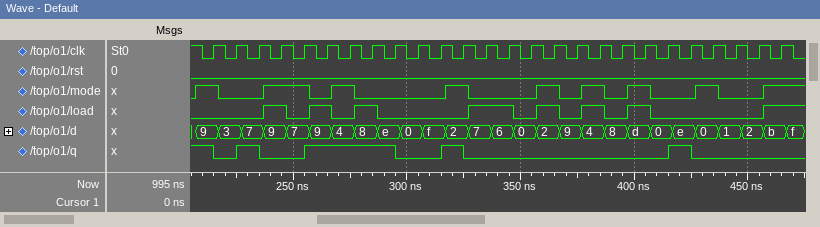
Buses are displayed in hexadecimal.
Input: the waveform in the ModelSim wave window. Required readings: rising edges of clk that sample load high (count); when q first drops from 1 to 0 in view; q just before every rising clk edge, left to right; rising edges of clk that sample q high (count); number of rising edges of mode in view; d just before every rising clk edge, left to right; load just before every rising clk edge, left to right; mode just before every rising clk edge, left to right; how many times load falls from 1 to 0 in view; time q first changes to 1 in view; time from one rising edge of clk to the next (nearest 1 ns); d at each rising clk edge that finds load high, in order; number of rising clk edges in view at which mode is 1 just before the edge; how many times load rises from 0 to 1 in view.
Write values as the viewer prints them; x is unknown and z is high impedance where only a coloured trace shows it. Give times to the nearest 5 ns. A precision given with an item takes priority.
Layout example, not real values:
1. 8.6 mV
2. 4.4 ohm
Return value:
1. 9
2. 215 ns
3. 1 0 1 0 0 1 1 1 1 0 0 1 0 0 0 0 0 0 0 0 0 1 0 0 0 0
4. 8
5. 9
6. 9, 3, 7, 9, 7, 9, 4, 8, e, 0, f, 2, 7, 6, 0, 2, 9, 4, 8, d, 0, e, 0, 1, 2, b
7. 0 0 0 1 0 1 0 1 0 0 0 0 1 1 0 1 0 1 0 1 0 0 0 0 0 1
8. 1 0 0 1 1 0 1 0 0 0 0 1 0 0 0 1 0 1 0 1 0 0 1 0 0 1
9. 7
10. 225 ns
11. 10 ns
12. 9, 9, 8, 7, 6, 2, 4, d, b
13. 10
14. 8
